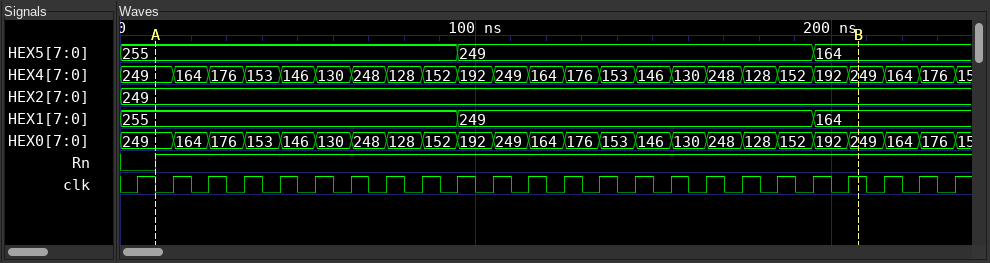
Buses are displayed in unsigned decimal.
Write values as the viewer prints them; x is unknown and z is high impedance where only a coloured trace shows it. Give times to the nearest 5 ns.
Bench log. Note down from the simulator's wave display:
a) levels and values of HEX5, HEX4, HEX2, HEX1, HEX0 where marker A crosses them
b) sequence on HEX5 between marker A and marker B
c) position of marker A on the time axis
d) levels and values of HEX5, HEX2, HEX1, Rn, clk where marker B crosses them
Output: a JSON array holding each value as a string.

["HEX5=255, HEX4=249, HEX2=249, HEX1=255, HEX0=249", "255, 249, 164", "10 ns", "HEX5=164, HEX2=249, HEX1=164, Rn=1, clk=1"]
